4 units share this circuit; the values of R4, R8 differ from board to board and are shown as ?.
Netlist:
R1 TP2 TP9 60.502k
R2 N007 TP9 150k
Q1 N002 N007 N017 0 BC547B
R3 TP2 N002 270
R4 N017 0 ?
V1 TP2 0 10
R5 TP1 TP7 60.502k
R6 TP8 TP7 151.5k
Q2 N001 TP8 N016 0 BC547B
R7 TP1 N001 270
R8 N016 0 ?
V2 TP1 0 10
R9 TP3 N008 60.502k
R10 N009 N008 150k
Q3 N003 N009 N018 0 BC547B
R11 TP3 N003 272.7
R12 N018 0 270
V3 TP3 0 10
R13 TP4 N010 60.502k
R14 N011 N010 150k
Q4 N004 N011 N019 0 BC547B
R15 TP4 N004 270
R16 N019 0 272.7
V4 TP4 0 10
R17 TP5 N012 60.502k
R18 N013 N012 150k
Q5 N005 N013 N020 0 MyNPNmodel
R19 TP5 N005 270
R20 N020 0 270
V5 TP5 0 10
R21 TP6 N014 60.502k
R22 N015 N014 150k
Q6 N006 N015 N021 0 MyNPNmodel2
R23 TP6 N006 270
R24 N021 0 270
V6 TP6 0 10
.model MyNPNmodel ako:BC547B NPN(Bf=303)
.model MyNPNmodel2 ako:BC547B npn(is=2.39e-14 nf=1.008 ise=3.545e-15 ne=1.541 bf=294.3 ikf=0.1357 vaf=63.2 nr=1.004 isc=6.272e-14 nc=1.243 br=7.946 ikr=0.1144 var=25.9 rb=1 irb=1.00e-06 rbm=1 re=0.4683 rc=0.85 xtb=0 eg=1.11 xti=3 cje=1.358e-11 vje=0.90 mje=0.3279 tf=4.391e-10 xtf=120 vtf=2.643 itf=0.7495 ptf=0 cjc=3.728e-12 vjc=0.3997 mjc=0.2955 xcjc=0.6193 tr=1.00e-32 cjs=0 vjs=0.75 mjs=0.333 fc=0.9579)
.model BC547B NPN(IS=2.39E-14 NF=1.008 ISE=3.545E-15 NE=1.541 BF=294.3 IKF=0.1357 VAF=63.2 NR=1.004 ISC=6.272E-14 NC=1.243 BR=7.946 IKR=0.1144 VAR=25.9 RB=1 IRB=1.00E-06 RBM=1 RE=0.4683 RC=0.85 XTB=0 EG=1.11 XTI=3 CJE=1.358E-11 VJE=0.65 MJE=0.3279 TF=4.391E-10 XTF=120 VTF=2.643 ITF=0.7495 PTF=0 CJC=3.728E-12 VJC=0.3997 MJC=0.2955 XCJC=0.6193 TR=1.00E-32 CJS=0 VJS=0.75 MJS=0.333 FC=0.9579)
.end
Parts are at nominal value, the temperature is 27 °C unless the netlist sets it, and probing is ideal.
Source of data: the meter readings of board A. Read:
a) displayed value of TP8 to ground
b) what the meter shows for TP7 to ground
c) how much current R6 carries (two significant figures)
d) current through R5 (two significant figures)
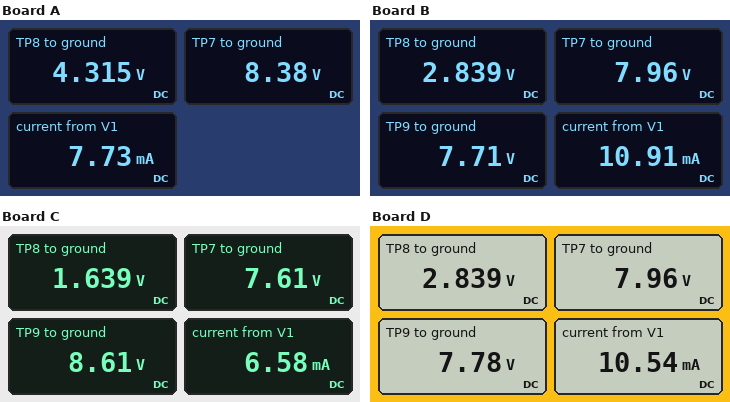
4.315 V
8.38 V
27 µA
27 µA
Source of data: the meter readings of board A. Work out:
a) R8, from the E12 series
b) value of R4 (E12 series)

470 Ω
470 Ω
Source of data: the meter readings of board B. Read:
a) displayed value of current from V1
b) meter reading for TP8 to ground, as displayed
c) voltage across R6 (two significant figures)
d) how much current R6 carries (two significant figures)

10.91 mA
2.839 V
5.1 V
34 µA
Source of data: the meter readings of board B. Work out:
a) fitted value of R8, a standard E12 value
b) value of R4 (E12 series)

220 Ω
120 Ω
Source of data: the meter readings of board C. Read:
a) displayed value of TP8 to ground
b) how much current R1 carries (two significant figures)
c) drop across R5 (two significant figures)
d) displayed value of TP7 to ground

1.639 V
23 µA
2.4 V
7.61 V
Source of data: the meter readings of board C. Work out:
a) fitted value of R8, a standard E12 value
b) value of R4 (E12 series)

82 Ω
680 Ω
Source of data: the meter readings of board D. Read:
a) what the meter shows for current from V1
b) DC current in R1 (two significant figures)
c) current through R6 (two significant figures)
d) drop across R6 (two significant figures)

10.54 mA
37 µA
34 µA
5.1 V
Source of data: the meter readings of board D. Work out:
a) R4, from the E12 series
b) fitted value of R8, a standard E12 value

150 Ω
220 Ω
